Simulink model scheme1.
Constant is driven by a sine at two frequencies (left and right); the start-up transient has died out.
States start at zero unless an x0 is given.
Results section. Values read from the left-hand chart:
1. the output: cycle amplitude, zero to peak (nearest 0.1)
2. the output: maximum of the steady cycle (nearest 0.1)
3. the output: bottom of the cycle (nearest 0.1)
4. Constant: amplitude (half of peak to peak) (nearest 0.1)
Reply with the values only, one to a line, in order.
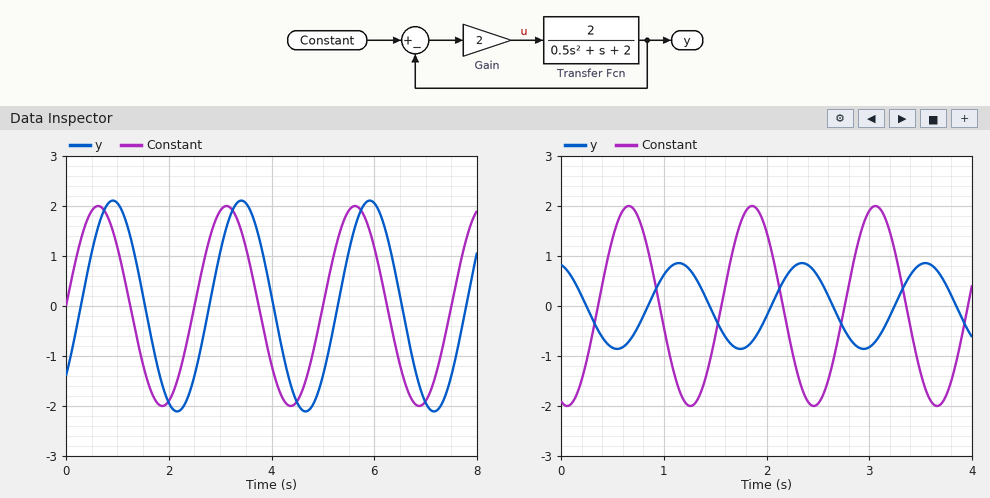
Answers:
2.1
2.1
-2.1
2.0
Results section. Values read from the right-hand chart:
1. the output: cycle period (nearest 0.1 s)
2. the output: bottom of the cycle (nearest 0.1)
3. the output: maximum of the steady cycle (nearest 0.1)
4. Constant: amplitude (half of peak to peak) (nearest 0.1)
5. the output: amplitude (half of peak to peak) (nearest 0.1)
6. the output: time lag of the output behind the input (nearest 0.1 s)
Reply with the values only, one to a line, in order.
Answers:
1.2 s
-0.9
0.9
2.0
0.9
0.5 s
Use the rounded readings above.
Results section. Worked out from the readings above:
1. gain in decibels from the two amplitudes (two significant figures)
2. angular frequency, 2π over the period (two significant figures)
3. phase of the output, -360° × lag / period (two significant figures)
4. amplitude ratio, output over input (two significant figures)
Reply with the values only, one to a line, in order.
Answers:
-6.9 dB
5.2 rad/s
-150°
0.45
